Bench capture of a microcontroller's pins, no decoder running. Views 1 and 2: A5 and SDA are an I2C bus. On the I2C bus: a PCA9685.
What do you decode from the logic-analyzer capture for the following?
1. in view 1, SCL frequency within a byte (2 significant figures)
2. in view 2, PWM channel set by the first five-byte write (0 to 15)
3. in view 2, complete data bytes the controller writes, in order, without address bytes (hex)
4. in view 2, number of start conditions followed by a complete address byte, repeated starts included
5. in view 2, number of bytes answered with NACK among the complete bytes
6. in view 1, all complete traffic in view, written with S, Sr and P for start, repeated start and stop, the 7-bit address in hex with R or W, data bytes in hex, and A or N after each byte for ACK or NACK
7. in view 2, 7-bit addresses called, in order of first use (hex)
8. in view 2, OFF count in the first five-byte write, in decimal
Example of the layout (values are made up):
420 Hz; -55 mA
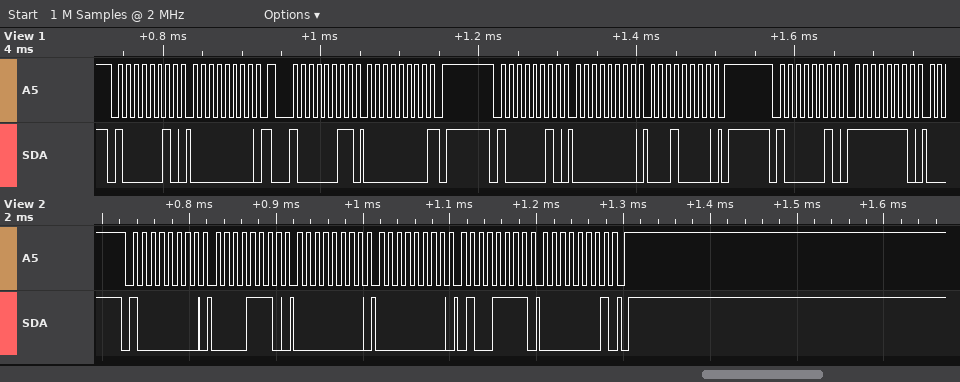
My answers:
100 kHz; 2; 0E 00 00 4F 01; 1; 0; S 41W A 00 A Sr 41R A 00 N P S 41W A 00 A 10 A P S 41W A FE A; 0x40; 335
